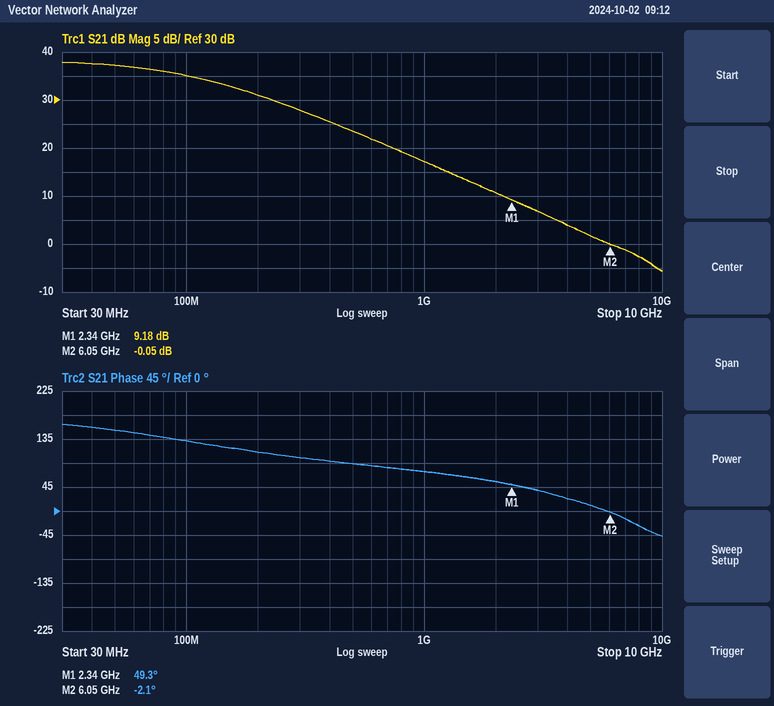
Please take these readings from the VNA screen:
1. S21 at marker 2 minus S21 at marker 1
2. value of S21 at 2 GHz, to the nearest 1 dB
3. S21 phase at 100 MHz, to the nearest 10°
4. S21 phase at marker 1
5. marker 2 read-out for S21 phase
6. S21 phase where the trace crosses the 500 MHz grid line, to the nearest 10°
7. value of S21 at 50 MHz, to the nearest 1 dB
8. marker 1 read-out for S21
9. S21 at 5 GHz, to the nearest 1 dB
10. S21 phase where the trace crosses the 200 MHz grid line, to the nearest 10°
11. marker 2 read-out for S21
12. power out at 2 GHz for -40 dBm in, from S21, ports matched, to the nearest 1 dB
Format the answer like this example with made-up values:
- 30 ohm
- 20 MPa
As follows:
- -9.23 dB
- 11 dB
- 130°
- 49.3°
- -2.1°
- 90°
- 37 dB
- 9.18 dB
- 2 dB
- 110°
- -0.05 dB
- -29 dBm
